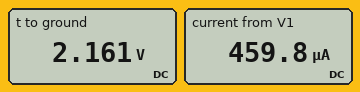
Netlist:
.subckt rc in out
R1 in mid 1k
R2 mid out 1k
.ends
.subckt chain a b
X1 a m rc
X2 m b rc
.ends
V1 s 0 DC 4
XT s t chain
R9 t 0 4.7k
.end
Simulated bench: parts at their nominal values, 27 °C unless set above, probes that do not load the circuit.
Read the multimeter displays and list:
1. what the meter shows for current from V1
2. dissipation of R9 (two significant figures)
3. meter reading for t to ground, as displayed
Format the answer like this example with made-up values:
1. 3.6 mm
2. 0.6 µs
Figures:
1. 459.8 µA
2. 990 µW
3. 2.161 V
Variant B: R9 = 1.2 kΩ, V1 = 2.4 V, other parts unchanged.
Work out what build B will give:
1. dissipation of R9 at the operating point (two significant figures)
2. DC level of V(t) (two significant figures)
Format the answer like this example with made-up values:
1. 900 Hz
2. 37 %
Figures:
1. 260 µW
2. 550 mV
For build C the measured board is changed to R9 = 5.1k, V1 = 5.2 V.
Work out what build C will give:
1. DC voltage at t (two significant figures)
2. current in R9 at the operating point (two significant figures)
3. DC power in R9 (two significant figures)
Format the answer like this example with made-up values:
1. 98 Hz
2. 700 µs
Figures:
1. 2.9 V
2. 570 µA
3. 1.7 mW
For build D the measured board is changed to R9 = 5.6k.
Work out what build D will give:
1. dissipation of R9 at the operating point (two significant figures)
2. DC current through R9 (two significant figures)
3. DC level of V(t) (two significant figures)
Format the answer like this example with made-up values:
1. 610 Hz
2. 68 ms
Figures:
1. 970 µW
2. 420 µA
3. 2.3 V
